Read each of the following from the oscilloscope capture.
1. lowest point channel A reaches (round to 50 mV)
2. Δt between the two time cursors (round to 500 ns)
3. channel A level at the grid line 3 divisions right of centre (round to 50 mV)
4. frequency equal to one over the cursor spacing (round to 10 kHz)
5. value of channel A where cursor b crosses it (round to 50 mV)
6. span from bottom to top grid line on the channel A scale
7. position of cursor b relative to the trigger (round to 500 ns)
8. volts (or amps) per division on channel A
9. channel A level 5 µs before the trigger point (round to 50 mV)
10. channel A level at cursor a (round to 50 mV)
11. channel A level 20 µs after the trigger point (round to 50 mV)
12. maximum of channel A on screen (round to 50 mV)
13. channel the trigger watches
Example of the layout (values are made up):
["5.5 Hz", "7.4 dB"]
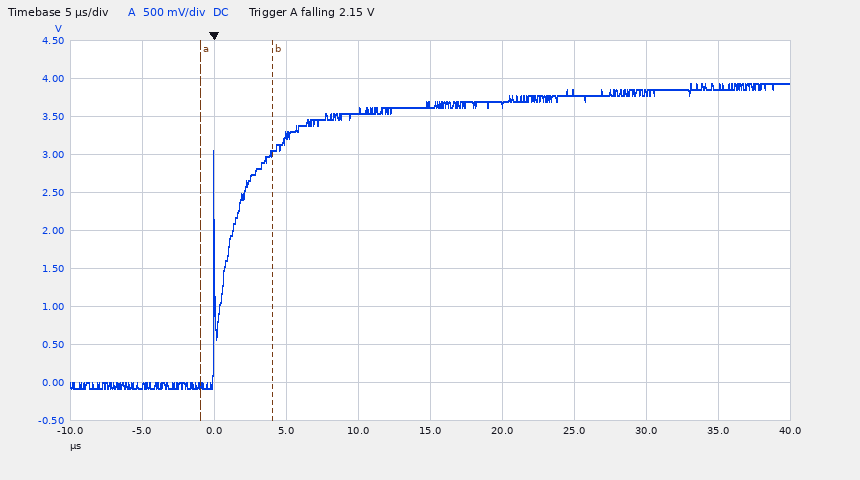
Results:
["-100 mV", "5.0 µs", "3.80 V", "200 kHz", "3.00 V", "5 V", "+4.0 µs", "500 mV", "-50 mV", "-50 mV", "3.65 V", "3.95 V", "channel A"]
